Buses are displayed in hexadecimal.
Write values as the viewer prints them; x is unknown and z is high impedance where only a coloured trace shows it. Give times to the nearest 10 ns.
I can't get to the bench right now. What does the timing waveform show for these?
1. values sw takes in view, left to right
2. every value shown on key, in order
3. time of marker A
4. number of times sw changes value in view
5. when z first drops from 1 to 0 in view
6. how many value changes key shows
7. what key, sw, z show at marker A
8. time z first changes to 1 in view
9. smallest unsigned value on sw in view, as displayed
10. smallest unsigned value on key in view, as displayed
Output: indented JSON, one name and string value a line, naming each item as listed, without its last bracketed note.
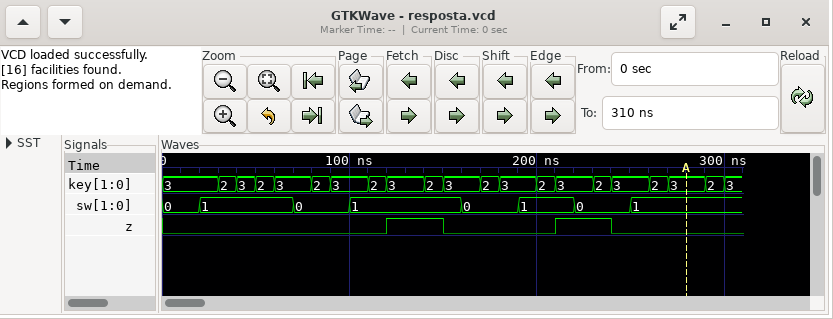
{
  "values sw takes in view, left to right": "0, 1, 0, 1, 0, 1, 0, 1",
  "every value shown on key, in order": "3, 2, 3, 2, 3, 2, 3, 2, 3, 2, 3, 2, 3, 2, 3, 2, 3, 2, 3, 2, 3",
  "time of marker A": "280 ns",
  "number of times sw changes value in view": "7",
  "when z first drops from 1 to 0 in view": "150 ns",
  "how many value changes key shows": "20",
  "what key, sw, z show at marker A": "key=3, sw=1, z=0",
  "time z first changes to 1 in view": "120 ns",
  "smallest unsigned value on sw in view, as displayed": "0",
  "smallest unsigned value on key in view, as displayed": "2"
}
